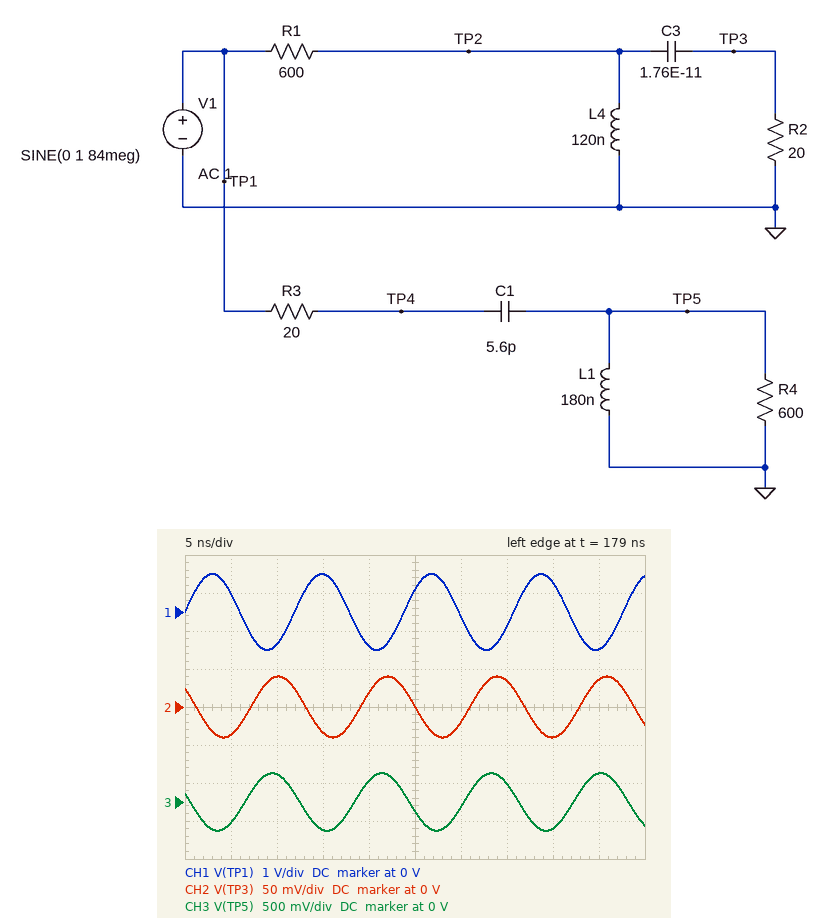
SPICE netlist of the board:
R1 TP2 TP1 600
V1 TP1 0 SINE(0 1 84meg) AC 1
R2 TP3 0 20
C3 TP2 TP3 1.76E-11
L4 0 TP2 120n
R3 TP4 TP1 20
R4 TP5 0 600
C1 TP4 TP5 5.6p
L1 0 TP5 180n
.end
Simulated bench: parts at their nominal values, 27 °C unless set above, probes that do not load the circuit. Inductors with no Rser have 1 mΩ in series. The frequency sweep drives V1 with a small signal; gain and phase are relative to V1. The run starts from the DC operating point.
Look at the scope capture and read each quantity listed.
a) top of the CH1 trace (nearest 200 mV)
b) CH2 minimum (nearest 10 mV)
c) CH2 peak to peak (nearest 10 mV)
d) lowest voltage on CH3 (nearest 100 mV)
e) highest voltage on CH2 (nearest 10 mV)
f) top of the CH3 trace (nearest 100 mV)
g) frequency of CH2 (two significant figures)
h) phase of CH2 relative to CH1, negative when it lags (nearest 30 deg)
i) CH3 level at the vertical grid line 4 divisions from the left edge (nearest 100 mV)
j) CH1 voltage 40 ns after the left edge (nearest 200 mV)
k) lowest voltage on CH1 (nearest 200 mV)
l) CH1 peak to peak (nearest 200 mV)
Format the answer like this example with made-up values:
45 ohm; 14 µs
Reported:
1.0 V; -40 mV; 80 mV; -400 mV; 40 mV; 400 mV; 84 MHz; 150 deg; 300 mV; 800 mV; -1.0 V; 2.0 V
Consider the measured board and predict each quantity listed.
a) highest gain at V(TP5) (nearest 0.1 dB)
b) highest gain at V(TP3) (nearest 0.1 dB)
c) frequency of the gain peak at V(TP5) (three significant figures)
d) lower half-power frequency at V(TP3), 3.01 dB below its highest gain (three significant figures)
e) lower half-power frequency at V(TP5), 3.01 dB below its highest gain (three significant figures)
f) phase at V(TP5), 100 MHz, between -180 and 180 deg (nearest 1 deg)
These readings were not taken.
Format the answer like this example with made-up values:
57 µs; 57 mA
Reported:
7.8 dB; -21.1 dB; 163 MHz; 94.6 MHz; 136 MHz; 156 deg
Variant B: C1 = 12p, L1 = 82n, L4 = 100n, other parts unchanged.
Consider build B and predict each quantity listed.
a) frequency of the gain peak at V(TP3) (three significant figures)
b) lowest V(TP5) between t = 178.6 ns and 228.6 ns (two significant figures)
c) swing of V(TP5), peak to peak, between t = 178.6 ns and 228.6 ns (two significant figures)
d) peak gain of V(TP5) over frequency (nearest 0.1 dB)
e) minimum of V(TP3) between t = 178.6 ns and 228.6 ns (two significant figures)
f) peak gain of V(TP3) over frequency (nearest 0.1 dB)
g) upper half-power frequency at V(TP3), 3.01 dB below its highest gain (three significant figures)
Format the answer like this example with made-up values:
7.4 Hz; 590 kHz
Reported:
123 MHz; -370 mV; 740 mV; 8.4 dB; -29 mV; -21.4 dB; 159 MHz
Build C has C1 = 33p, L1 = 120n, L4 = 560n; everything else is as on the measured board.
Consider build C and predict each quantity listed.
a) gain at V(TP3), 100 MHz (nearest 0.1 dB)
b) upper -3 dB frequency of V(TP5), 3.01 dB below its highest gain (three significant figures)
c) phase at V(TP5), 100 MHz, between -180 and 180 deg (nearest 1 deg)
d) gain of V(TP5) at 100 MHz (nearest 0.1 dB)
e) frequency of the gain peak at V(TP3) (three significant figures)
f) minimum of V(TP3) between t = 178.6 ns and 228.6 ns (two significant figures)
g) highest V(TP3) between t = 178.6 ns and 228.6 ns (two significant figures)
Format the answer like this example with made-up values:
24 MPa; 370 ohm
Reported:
-27.6 dB; 112 MHz; 41 deg; 5.6 dB; 52.0 MHz; -47 mV; 47 mV
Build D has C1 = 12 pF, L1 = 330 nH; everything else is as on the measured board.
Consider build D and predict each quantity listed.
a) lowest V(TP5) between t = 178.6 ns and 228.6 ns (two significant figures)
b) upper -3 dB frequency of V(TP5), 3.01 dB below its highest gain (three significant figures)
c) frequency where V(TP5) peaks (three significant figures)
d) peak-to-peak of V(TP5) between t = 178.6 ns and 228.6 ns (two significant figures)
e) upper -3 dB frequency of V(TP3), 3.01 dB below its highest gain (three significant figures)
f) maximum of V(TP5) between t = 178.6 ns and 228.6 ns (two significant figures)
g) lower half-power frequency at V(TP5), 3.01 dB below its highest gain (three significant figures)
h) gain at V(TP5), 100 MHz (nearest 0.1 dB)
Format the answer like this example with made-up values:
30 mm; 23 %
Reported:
-2.5 V; 107 MHz; 81.9 MHz; 5.0 V; 144 MHz; 2.5 V; 68.8 MHz; 5.9 dB
